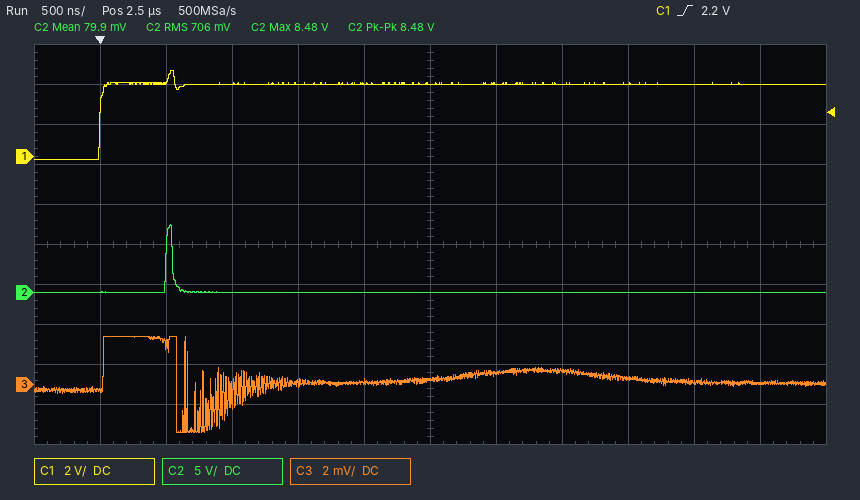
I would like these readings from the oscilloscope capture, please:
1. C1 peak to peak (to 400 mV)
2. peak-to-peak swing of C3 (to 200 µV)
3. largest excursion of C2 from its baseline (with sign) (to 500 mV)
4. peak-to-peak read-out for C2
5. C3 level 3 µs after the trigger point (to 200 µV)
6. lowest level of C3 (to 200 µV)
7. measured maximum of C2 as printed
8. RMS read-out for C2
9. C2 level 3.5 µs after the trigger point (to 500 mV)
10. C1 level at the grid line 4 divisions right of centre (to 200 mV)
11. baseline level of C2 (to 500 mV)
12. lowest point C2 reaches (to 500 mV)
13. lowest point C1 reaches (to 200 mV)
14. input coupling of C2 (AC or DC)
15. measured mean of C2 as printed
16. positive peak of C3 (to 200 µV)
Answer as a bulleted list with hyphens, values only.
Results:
- 4.4 V
- 4.8 mV
- +8.5 V
- 8.48 V
- 600 µV
- -2.4 mV
- 8.48 V
- 706 mV
- 0.0 V
- 3.6 V
- 0.0 V
- 0.0 V
- -200 mV
- DC
- 79.9 mV
- 2.4 mV
